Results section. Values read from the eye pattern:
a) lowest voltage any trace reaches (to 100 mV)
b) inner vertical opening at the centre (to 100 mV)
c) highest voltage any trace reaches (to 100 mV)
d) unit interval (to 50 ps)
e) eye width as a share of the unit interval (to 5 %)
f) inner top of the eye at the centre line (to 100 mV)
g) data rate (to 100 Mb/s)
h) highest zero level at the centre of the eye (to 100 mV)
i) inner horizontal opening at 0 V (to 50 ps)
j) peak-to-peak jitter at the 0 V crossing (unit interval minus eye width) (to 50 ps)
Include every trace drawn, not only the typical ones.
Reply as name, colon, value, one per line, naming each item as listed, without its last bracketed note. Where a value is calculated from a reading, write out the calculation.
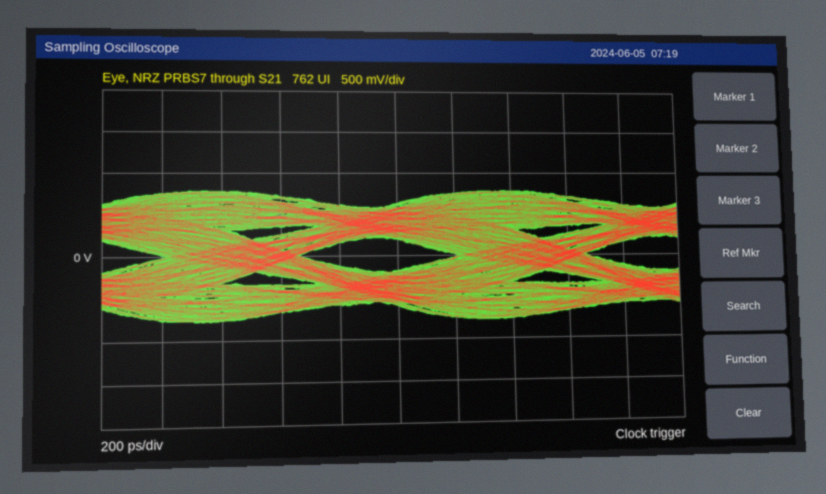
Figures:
lowest voltage any trace reaches: -800 mV
inner vertical opening at the centre: 400 mV
highest voltage any trace reaches: 800 mV
unit interval: 1.00 ns
eye width as a share of the unit interval: 550 ps / 1.00 ns ≈ 55 %
inner top of the eye at the centre line: 200 mV
data rate: 1.0 Gb/s
highest zero level at the centre of the eye: -200 mV
inner horizontal opening at 0 V: 550 ps
peak-to-peak jitter at the 0 V crossing (unit interval minus eye width): 450 ps
